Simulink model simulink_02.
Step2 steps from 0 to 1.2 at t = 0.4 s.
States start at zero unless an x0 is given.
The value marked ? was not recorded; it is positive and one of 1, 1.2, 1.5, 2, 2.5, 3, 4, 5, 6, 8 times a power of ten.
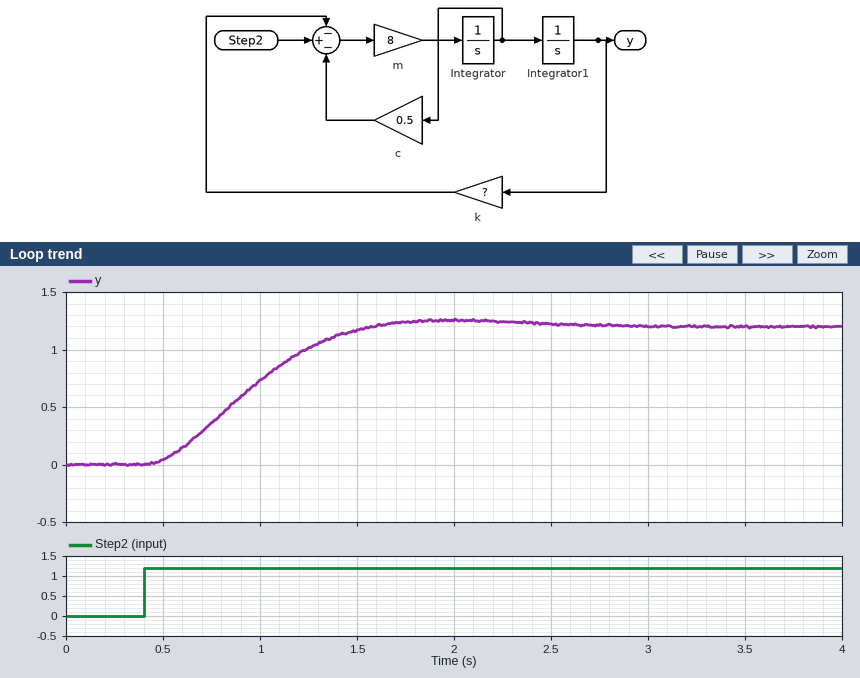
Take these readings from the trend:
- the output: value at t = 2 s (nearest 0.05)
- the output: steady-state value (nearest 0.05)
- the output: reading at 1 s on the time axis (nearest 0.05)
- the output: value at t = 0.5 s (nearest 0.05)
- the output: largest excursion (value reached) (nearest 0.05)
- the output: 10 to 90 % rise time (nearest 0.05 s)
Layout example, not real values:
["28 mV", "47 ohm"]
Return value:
["1.25", "1.20", "0.75", "0.05", "1.25", "0.75 s"]
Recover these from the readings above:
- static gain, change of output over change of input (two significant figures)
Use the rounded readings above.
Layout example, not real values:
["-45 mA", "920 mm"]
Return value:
["1.0"]
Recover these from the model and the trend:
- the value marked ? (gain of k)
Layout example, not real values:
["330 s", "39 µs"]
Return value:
["1"]
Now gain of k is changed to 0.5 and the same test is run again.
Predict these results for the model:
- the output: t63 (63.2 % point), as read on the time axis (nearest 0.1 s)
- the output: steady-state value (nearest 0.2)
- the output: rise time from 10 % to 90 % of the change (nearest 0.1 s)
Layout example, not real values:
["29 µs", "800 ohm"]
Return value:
["1.5 s", "2.4", "1.7 s"]
